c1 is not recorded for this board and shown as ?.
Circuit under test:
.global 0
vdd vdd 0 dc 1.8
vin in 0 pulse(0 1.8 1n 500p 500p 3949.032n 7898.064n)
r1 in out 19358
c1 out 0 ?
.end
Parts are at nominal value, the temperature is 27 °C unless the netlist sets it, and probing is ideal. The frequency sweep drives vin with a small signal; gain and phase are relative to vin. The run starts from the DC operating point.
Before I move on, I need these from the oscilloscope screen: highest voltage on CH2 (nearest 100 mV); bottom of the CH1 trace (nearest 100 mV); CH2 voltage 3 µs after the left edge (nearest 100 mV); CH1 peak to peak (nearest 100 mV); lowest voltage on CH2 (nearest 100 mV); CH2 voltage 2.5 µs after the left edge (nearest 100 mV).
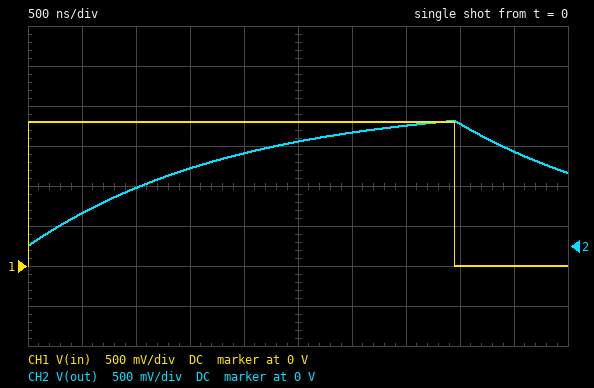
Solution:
1.6 V
0 V
1.4 V
1.8 V
0 V
1.3 V
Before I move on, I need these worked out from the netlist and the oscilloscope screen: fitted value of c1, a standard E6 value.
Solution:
100 pF
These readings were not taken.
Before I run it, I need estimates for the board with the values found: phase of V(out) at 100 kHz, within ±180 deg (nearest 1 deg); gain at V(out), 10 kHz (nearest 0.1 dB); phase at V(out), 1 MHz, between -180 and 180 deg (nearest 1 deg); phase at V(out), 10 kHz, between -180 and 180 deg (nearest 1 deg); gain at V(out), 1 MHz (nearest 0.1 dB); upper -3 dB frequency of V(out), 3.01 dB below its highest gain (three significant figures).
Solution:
-51 deg
-0.1 dB
-85 deg
-7 deg
-21.7 dB
82.2 kHz
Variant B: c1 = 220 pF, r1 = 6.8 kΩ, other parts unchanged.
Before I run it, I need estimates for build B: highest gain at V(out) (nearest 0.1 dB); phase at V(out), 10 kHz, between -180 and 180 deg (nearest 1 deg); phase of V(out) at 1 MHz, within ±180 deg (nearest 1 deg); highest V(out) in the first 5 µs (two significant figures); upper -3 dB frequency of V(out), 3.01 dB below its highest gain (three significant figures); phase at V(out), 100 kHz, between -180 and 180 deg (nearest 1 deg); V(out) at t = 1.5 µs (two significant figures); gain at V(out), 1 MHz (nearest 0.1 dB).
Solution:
0 dB
-5 deg
-84 deg
1.7 V
106 kHz
-43 deg
1.1 V
-19.5 dB
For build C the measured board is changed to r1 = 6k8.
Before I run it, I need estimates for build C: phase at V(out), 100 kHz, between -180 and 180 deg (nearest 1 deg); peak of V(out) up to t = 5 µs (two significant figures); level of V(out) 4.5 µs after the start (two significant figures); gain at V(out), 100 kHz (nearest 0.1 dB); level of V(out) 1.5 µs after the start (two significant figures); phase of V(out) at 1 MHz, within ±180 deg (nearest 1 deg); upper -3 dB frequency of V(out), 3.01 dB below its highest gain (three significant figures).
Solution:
-23 deg
1.8 V
800 mV
-0.7 dB
1.6 V
-77 deg
234 kHz
